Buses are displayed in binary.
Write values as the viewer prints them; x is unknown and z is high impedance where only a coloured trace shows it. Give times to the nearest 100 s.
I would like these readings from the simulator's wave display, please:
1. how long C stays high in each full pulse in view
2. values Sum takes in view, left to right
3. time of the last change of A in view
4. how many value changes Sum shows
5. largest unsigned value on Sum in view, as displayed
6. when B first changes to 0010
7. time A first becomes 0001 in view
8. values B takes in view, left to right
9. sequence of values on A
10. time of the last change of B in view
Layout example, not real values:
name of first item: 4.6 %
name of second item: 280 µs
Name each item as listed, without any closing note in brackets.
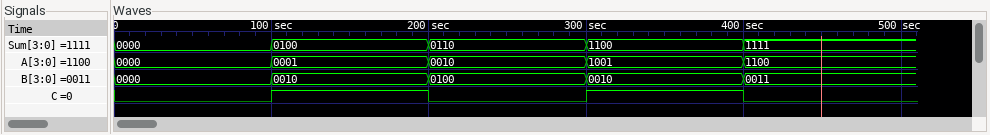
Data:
how long C stays high in each full pulse in view: 100 s, 100 s
values Sum takes in view, left to right: 0000, 0100, 0110, 1100, 1111
time of the last change of A in view: 400 s
how many value changes Sum shows: 4
largest unsigned value on Sum in view, as displayed: 1111
when B first changes to 0010: 100 s
time A first becomes 0001 in view: 100 s
values B takes in view, left to right: 0000, 0010, 0100, 0010, 0011
sequence of values on A: 0000, 0001, 0010, 1001, 1100
time of the last change of B in view: 400 s
